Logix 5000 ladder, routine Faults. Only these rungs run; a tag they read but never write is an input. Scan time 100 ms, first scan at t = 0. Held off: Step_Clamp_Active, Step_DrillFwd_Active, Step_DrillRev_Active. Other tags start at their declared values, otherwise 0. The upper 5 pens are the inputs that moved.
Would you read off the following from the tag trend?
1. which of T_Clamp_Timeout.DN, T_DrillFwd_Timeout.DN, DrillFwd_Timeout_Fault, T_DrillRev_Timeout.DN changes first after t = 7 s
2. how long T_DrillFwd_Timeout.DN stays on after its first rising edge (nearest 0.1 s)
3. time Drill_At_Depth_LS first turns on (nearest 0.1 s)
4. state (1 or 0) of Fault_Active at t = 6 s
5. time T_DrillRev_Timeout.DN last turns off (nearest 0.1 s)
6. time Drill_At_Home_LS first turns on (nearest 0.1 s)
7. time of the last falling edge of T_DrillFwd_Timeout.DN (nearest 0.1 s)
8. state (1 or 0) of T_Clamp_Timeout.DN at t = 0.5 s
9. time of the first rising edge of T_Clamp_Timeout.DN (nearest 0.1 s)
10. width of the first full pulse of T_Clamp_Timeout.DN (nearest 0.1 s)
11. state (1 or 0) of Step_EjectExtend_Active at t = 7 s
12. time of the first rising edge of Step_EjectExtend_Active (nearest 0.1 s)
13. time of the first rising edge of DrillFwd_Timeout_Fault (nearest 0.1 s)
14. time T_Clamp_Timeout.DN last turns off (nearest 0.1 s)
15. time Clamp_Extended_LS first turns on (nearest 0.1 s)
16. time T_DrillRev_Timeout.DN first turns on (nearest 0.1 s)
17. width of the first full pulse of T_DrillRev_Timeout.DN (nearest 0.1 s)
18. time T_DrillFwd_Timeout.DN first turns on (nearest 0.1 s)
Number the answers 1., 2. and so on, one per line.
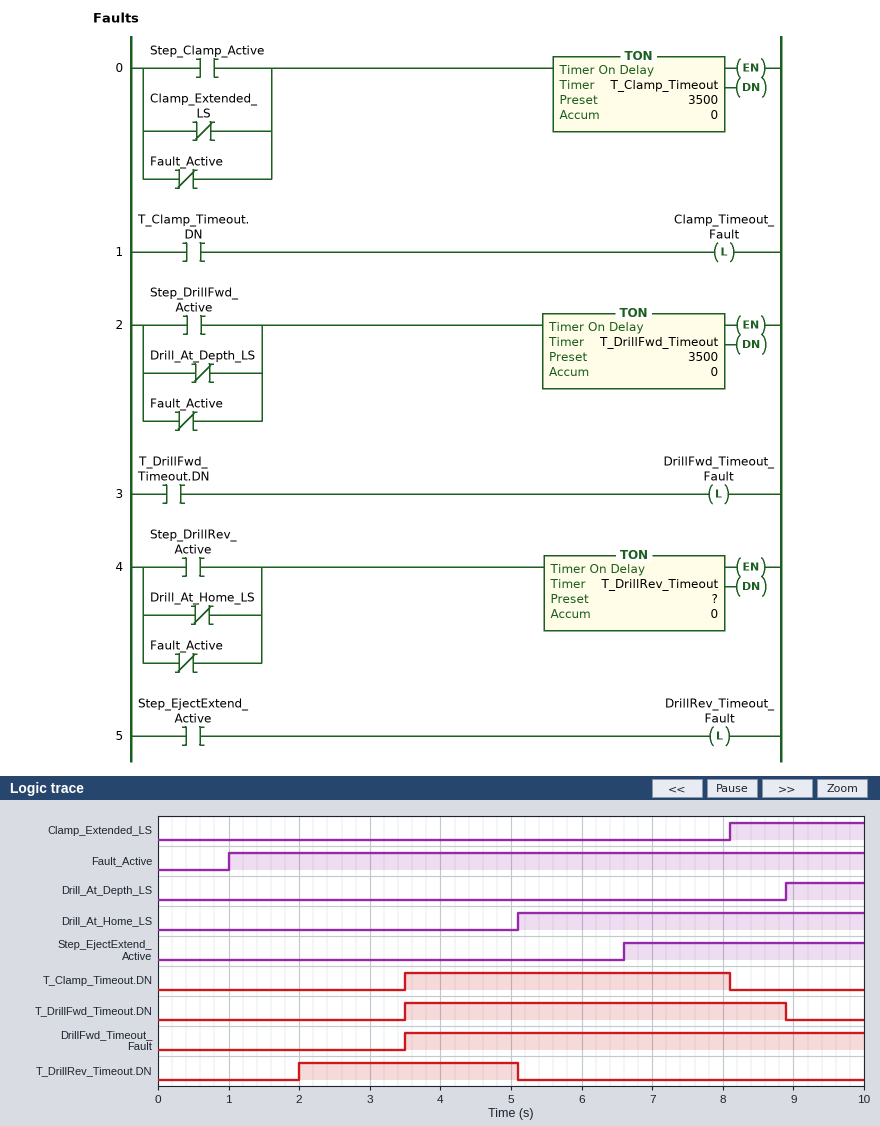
1. T_Clamp_Timeout.DN
2. 5.4 s
3. 8.9 s
4. 1
5. 5.1 s
6. 5.1 s
7. 8.9 s
8. 0
9. 3.5 s
10. 4.6 s
11. 1
12. 6.6 s
13. 3.5 s
14. 8.1 s
15. 8.1 s
16. 2.0 s
17. 3.1 s
18. 3.5 s
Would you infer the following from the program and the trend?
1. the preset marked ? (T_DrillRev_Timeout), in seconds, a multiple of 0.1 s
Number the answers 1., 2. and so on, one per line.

1. 2.0 s
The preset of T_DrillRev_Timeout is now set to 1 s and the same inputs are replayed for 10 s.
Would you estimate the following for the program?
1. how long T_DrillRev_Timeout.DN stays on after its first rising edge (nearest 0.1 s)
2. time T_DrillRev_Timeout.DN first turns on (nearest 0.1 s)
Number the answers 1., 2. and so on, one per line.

1. 4.1 s
2. 1.0 s
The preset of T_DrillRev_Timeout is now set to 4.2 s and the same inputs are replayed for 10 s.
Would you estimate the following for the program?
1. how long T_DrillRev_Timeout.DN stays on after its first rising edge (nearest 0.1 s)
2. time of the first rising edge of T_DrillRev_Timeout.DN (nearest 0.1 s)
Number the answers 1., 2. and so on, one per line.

1. 0.9 s
2. 4.2 s
